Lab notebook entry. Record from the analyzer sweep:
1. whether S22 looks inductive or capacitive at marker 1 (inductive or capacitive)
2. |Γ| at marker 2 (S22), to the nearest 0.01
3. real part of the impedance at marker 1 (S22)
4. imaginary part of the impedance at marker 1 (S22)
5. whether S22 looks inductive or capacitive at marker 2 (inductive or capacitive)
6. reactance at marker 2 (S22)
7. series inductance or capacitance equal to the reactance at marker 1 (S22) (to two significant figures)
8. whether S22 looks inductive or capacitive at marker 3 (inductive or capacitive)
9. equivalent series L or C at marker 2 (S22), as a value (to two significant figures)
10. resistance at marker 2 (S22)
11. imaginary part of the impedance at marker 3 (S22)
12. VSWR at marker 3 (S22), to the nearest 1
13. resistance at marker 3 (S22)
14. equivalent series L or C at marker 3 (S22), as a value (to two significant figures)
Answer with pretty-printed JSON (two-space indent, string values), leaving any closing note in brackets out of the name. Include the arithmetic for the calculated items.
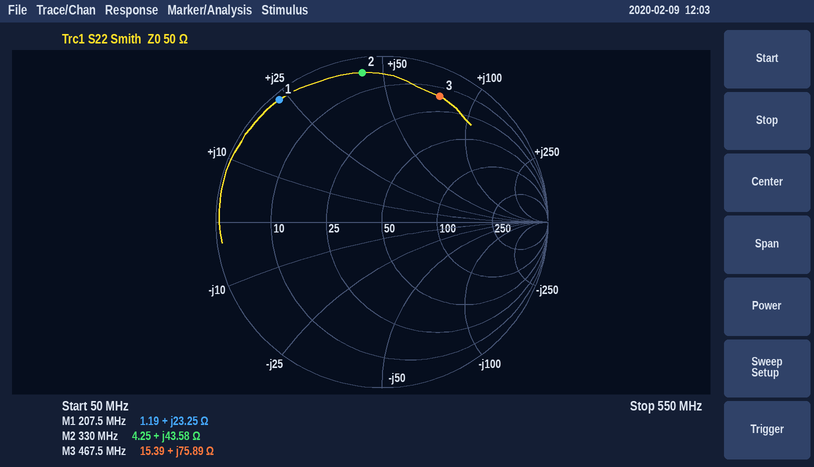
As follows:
{
  "whether S22 looks inductive or capacitive at marker 1": "inductive",
  "|Γ| at marker 2 (S22), to the nearest 0.01": "0.91",
  "real part of the impedance at marker 1": "1.19 Ω",
  "imaginary part of the impedance at marker 1": "+23.25 Ω",
  "whether S22 looks inductive or capacitive at marker 2": "inductive",
  "reactance at marker 2": "+43.58 Ω",
  "series inductance or capacitance equal to the reactance at marker 1 (S22)": "L = 23.25 Ω/(2π × 207.5 MHz) ≈ 18 nH",
  "whether S22 looks inductive or capacitive at marker 3": "inductive",
  "equivalent series L or C at marker 2 (S22), as a value": "L = 43.58 Ω/(2π × 330 MHz) ≈ 21 nH",
  "resistance at marker 2": "4.25 Ω",
  "imaginary part of the impedance at marker 3": "+75.89 Ω",
  "VSWR at marker 3 (S22), to the nearest 1": "11",
  "resistance at marker 3": "15.39 Ω",
  "equivalent series L or C at marker 3 (S22), as a value": "L = 75.89 Ω/(2π × 467.5 MHz) ≈ 26 nH"
}
